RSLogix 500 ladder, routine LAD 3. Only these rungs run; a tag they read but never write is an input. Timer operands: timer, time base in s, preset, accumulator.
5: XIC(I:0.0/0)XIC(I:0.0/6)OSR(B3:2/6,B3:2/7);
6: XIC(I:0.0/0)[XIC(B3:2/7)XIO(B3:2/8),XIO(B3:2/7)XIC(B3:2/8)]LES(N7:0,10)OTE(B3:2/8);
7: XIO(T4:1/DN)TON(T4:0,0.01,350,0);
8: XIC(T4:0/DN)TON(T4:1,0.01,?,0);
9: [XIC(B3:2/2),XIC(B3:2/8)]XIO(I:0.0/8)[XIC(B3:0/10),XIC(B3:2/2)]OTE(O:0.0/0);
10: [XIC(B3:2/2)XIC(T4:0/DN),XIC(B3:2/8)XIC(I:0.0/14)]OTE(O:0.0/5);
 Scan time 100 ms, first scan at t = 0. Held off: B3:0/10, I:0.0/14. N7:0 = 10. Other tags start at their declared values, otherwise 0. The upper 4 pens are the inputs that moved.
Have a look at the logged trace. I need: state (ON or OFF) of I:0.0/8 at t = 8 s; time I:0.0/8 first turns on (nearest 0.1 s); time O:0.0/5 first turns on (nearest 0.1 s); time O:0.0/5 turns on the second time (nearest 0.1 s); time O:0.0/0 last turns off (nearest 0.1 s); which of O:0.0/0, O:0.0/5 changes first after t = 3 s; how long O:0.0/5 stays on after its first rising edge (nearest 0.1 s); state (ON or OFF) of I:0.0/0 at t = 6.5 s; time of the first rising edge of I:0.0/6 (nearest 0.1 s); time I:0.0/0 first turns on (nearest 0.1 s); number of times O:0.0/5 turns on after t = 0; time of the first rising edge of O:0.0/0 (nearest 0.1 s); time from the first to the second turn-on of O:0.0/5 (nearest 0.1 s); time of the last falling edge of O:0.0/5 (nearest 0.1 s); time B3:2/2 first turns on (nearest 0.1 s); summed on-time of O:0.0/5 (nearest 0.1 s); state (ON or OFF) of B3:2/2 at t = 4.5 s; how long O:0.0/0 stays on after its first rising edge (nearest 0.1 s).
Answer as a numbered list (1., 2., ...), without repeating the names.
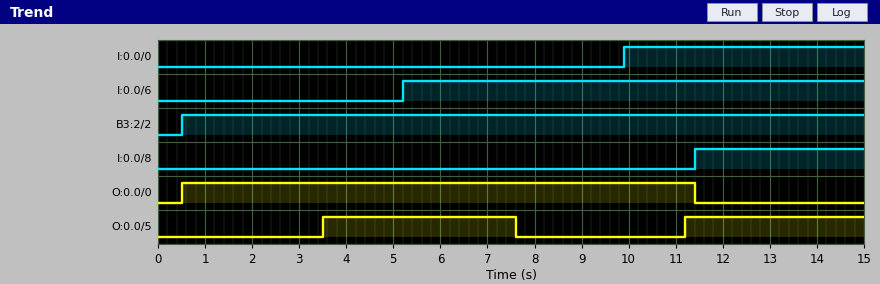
1. OFF
2. 11.4 s
3. 3.5 s
4. 11.2 s
5. 11.4 s
6. O:0.0/5
7. 4.1 s
8. OFF
9. 5.2 s
10. 9.9 s
11. 2
12. 0.5 s
13. 7.7 s
14. 7.6 s
15. 0.5 s
16. 7.9 s
17. ON
18. 10.9 s
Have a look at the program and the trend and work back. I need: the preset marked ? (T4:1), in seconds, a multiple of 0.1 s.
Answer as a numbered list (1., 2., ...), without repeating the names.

1. 4.0 s
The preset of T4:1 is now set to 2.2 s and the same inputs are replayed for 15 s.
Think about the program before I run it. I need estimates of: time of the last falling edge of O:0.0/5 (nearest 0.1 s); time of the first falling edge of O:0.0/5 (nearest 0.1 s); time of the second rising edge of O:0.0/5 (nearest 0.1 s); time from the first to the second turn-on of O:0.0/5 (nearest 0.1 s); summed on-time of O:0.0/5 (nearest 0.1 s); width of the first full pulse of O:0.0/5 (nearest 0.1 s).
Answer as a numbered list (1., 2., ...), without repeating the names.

1. 11.7 s
2. 5.8 s
3. 9.4 s
4. 5.9 s
5. 4.6 s
6. 2.3 s
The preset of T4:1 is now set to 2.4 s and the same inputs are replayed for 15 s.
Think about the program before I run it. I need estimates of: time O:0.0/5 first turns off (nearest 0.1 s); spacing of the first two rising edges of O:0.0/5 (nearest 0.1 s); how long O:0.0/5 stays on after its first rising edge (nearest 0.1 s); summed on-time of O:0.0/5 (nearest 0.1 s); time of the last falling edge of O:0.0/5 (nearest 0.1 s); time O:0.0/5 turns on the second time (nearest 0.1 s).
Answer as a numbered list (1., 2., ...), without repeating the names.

1. 6.0 s
2. 6.1 s
3. 2.5 s
4. 5.0 s
5. 12.1 s
6. 9.6 s
